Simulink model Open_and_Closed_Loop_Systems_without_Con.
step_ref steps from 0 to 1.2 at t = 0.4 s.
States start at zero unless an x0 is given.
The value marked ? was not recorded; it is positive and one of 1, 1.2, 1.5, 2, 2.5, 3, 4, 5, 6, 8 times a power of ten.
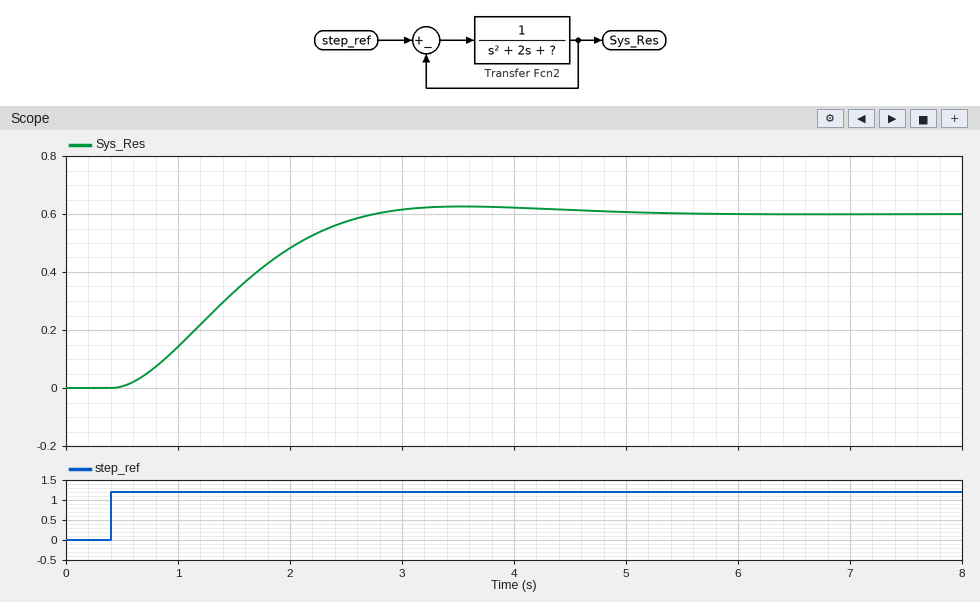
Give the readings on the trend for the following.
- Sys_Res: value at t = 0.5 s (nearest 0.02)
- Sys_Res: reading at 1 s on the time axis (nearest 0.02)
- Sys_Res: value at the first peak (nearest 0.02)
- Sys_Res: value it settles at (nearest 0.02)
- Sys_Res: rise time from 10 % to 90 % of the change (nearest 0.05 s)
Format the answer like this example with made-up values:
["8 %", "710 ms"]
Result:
["0.00", "0.14", "0.62", "0.60", "1.50 s"]
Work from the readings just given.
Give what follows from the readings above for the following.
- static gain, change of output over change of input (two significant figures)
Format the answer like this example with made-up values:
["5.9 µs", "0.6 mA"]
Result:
["0.50"]
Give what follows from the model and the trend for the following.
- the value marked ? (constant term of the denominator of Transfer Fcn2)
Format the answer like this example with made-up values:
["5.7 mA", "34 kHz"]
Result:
["1"]
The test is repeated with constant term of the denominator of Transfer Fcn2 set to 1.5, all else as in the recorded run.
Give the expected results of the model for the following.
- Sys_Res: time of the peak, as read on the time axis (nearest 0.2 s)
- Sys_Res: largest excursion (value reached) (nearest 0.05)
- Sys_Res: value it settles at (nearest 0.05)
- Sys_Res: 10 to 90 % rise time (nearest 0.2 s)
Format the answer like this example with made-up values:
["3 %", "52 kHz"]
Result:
["3.0 s", "0.50", "0.50", "1.2 s"]
